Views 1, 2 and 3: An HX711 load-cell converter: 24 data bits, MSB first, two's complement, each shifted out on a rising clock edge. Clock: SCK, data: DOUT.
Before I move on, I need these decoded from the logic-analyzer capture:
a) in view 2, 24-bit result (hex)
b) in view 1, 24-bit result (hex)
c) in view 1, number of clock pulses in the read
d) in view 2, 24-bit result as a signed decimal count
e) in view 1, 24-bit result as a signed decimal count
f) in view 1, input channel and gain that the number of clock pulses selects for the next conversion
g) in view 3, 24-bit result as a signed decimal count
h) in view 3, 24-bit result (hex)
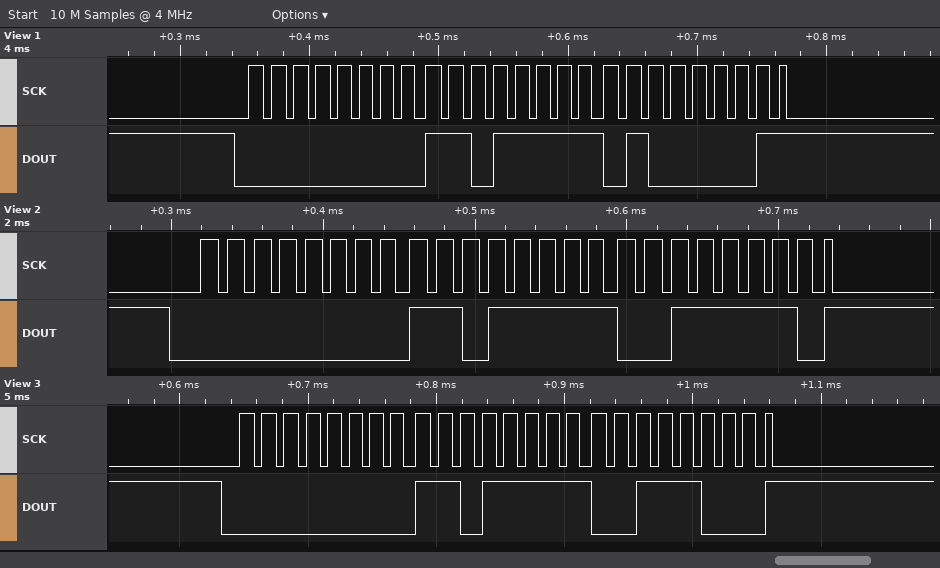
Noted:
0x00DF3E
0x00DF41
25
57150
57153
channel A, gain 128
57144
0x00DF38
